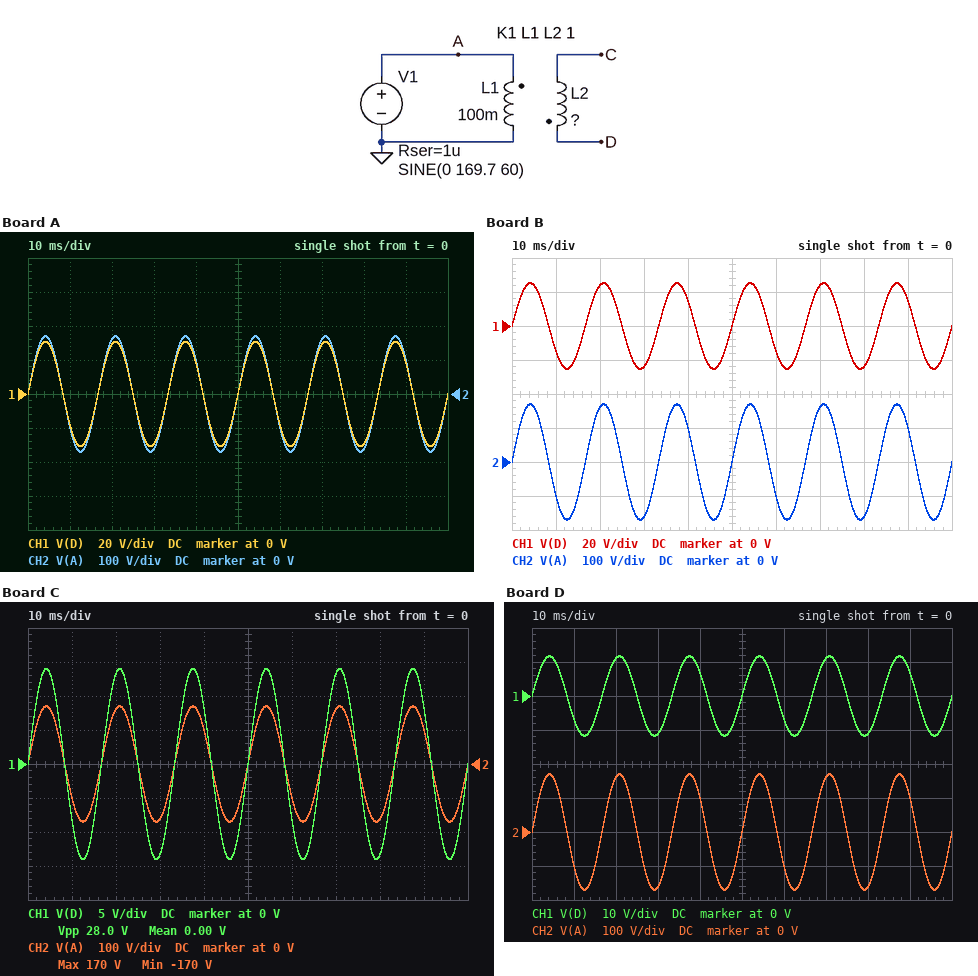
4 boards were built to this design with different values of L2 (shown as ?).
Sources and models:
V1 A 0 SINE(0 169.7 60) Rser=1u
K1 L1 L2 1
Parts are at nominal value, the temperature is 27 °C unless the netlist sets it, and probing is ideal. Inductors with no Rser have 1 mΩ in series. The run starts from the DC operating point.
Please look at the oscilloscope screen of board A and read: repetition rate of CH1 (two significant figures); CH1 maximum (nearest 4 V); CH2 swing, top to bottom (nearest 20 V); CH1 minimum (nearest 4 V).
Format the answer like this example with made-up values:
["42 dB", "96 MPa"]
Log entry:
["60 Hz", "32 V", "340 V", "-32 V"]
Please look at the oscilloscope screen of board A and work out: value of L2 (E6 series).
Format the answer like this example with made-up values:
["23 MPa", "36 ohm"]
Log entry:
["3.3 mH"]
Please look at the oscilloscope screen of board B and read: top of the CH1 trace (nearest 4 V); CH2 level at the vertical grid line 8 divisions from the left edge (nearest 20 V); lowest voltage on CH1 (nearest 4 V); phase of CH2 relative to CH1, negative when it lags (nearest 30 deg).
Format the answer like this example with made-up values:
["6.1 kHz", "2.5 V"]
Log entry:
["24 V", "-160 V", "-24 V", "0 deg"]
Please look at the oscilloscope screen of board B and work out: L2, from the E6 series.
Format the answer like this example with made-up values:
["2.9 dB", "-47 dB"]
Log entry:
["2.2 mH"]
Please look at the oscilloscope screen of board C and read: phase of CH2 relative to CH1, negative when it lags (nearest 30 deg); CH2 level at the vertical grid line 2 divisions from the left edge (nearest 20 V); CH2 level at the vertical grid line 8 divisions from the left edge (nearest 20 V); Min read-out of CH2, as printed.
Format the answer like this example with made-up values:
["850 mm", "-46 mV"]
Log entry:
["0 deg", "160 V", "-160 V", "-170 V"]
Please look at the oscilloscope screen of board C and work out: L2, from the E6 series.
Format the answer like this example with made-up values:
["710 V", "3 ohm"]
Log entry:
["680 µH"]
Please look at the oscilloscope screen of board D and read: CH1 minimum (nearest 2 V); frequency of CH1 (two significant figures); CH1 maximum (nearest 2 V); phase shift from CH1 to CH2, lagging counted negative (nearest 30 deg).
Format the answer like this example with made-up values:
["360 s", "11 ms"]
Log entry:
["-12 V", "60 Hz", "12 V", "0 deg"]
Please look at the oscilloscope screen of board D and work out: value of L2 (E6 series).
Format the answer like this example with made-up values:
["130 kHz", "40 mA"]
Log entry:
["470 µH"]
